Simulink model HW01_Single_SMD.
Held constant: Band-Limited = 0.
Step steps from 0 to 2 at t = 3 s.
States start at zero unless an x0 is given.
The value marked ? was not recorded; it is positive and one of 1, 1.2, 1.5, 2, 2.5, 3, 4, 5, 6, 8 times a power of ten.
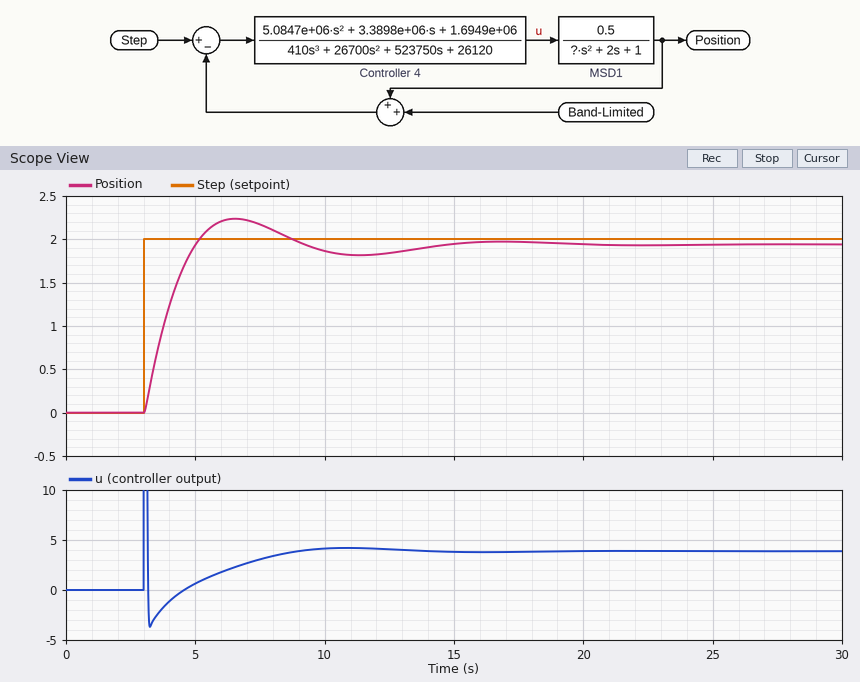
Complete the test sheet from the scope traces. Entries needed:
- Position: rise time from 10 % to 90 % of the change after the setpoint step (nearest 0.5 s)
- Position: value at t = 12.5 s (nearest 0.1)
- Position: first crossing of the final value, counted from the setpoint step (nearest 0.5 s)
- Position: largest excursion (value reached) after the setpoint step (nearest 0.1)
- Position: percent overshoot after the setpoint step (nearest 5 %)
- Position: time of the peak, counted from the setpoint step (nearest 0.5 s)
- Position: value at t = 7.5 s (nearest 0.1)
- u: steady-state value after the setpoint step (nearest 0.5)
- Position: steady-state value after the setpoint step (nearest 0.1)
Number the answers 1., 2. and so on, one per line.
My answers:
1. 1.5 s
2. 1.8
3. 2.0 s
4. 2.2
5. 15 %
6. 3.5 s
7. 2.2
8. 4.0
9. 1.9
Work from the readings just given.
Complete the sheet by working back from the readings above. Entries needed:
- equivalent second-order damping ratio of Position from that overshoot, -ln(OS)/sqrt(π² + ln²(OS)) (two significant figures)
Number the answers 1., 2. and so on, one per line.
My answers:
1. 0.52
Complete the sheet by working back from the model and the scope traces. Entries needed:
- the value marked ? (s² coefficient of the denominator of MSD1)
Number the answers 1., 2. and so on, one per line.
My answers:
1. 6
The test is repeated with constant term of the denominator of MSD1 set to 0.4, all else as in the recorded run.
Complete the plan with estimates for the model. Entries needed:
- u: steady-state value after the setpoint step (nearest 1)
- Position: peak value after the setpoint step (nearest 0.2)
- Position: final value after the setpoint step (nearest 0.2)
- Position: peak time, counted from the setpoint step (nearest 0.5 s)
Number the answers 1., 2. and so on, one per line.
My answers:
1. 2
2. 2.4
3. 2.0
4. 4.0 s
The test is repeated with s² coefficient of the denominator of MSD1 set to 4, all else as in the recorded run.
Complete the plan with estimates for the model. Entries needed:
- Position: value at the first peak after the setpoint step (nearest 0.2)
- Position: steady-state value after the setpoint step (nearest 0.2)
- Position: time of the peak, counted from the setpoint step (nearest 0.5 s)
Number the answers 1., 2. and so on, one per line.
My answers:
1. 2.0
2. 2.0
3. 3.0 s
